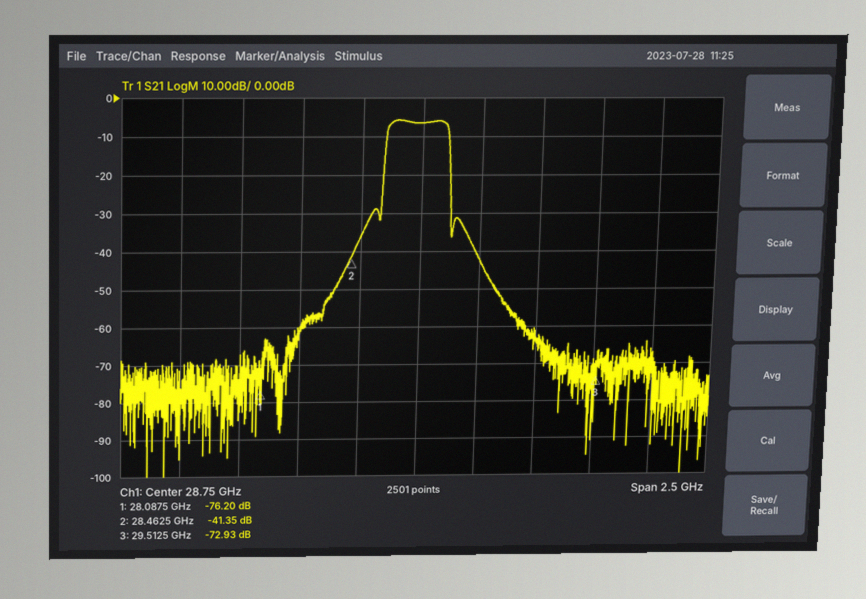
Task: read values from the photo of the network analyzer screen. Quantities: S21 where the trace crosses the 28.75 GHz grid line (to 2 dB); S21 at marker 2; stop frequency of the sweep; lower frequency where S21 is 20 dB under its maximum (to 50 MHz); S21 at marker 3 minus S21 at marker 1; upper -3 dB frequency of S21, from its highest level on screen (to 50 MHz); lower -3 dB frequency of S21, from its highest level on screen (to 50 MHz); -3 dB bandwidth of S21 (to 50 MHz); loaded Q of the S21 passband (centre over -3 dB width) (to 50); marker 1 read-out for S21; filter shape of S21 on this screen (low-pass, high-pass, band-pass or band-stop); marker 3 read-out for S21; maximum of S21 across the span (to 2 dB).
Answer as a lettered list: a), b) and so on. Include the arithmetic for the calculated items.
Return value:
a) -6 dB
b) -41.35 dB
c) 30 GHz
d) 28.60 GHz
e) -72.93 − (-76.2) = 3.27 dB
f) 28.85 GHz
g) 28.60 GHz
h) 28.85 GHz − 28.60 GHz = 250 MHz
i) 28.725 GHz / 250 MHz ≈ 115, so 100 to the nearest 50
j) -76.20 dB
k) band-pass
l) -72.93 dB
m) -6 dB
